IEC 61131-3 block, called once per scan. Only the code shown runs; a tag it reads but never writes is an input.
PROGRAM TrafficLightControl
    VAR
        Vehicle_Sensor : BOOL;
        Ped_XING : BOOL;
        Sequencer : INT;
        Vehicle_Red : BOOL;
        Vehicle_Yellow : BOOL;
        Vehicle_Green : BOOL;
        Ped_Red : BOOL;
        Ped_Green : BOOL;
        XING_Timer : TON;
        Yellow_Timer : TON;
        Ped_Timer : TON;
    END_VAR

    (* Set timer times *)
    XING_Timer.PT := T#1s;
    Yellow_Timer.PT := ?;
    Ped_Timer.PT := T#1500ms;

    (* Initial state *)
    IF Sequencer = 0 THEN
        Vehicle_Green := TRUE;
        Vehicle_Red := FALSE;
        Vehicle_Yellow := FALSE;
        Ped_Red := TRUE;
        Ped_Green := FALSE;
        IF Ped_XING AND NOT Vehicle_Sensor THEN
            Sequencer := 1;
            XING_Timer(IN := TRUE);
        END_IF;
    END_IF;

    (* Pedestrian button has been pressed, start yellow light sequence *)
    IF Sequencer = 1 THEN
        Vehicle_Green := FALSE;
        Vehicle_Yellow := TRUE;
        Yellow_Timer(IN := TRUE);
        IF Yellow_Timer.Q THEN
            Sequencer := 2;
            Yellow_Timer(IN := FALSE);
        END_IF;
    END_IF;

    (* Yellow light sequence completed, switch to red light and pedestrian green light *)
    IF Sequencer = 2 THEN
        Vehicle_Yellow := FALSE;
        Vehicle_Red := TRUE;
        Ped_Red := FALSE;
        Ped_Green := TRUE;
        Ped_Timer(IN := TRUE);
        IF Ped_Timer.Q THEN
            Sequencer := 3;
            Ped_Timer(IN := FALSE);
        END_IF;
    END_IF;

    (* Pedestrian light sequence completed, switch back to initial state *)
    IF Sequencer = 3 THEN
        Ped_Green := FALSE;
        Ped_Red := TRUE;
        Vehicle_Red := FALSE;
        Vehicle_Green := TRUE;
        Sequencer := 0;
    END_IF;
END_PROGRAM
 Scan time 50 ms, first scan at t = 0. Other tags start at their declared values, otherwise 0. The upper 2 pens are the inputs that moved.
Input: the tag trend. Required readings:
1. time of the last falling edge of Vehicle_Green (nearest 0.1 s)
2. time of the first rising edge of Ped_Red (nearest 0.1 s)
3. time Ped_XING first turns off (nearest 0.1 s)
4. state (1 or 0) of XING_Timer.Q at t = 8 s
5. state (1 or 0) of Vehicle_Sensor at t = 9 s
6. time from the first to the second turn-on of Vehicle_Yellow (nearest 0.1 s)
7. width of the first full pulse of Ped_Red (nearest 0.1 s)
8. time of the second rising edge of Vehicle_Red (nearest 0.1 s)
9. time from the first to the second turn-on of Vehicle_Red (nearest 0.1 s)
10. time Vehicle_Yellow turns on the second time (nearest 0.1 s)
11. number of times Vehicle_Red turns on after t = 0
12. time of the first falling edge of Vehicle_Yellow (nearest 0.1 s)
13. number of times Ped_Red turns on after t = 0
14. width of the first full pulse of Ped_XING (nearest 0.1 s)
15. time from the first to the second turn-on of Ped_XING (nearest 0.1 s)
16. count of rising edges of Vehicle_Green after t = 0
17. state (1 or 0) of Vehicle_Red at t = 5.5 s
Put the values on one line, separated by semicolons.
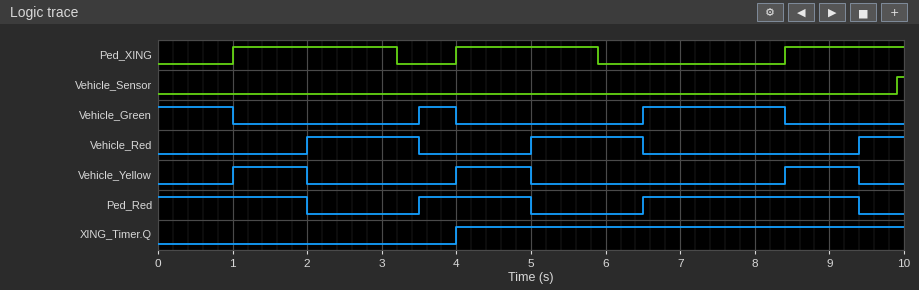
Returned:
8.4 s; 3.5 s; 3.2 s; 1; 0; 3.0 s; 1.5 s; 5.0 s; 3.0 s; 4.0 s; 3; 2.0 s; 2; 2.2 s; 3.0 s; 2; 1
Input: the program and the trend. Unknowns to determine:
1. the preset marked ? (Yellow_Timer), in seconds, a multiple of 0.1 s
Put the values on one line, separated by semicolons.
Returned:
1.0 s
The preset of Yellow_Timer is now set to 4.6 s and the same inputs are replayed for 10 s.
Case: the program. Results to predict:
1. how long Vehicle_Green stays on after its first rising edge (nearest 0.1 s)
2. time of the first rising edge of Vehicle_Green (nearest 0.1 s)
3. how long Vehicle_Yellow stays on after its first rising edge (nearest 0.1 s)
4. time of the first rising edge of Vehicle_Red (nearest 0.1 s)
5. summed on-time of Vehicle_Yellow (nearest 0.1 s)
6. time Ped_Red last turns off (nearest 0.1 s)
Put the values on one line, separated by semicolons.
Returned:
1.3 s; 7.1 s; 4.6 s; 5.6 s; 6.2 s; 5.6 s
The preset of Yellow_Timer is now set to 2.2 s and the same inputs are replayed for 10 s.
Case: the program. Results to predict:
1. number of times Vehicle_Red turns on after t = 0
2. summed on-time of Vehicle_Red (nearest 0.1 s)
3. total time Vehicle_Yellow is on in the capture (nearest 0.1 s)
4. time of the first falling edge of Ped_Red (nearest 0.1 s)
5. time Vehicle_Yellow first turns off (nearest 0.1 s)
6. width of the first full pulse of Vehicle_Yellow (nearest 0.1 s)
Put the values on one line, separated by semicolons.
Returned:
2; 3.0 s; 5.9 s; 3.2 s; 3.2 s; 2.2 s
